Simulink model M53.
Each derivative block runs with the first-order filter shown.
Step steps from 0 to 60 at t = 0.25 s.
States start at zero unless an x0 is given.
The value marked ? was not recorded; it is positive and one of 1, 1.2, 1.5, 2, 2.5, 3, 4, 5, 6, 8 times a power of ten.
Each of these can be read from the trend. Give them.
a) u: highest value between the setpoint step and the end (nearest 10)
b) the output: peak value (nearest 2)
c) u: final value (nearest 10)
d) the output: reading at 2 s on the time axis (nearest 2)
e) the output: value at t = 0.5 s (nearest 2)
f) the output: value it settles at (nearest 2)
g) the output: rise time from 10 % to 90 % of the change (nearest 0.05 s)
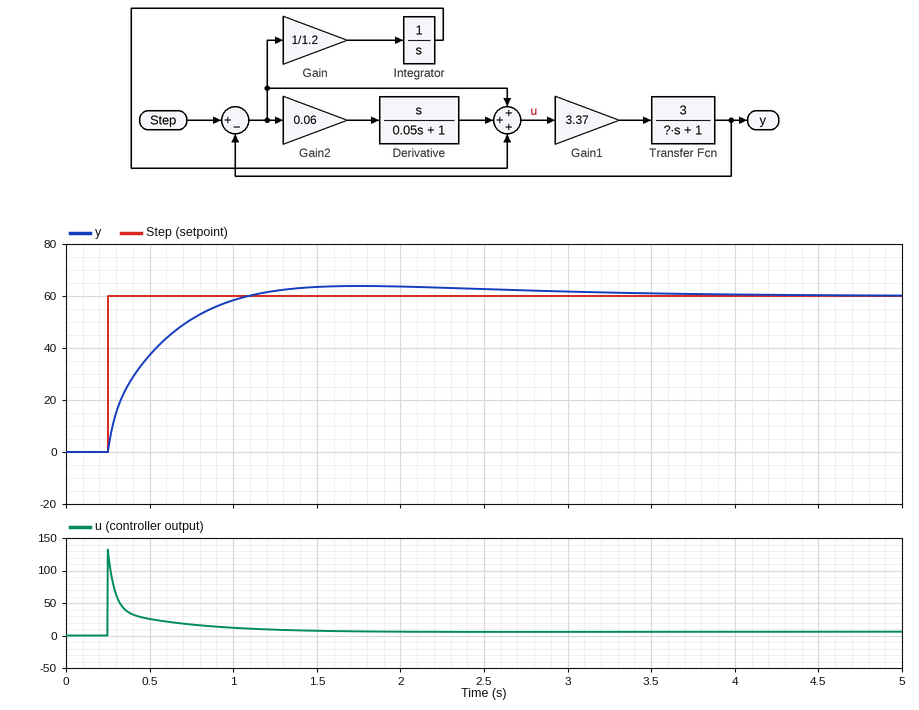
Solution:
130
64
10
64
38
60
0.55 s
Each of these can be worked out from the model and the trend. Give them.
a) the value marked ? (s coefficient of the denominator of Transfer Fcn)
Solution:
3
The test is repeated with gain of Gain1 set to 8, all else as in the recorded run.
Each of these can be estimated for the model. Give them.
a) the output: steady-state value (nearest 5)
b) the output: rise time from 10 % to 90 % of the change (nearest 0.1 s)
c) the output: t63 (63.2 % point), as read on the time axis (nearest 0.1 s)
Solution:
60
0.3 s
0.3 s
